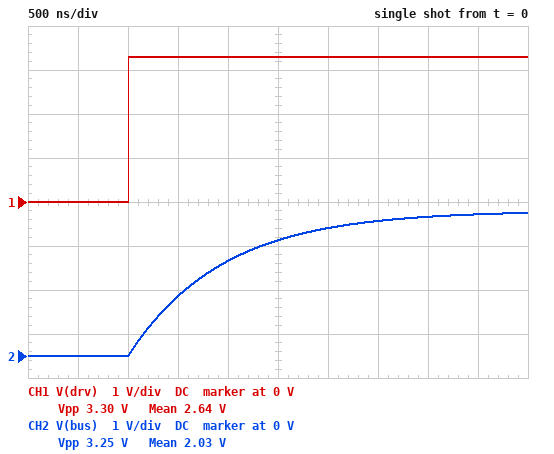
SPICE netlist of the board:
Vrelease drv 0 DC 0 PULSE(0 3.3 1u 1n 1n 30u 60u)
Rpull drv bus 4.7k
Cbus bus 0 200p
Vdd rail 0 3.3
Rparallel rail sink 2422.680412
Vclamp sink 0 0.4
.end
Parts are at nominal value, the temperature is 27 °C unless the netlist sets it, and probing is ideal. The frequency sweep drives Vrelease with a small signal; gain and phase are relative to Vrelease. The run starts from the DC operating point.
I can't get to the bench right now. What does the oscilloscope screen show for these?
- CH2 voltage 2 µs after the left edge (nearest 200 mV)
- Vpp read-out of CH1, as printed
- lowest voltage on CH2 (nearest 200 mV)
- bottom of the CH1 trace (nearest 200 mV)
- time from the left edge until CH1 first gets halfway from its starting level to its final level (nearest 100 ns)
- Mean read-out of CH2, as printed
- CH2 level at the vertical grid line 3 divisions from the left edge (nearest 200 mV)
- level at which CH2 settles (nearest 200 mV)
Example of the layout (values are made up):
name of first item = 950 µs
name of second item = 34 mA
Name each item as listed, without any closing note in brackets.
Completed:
CH2 voltage 2 µs after the left edge = 2.2 V
Vpp read-out of CH1, as printed = 3.30 V
lowest voltage on CH2 = 0 V
bottom of the CH1 trace = 0 V
time from the left edge until CH1 first gets halfway from its starting level to its final level = 1.0 µs
Mean read-out of CH2, as printed = 2.03 V
CH2 level at the vertical grid line 3 divisions from the left edge = 1.4 V
level at which CH2 settles = 3.2 V
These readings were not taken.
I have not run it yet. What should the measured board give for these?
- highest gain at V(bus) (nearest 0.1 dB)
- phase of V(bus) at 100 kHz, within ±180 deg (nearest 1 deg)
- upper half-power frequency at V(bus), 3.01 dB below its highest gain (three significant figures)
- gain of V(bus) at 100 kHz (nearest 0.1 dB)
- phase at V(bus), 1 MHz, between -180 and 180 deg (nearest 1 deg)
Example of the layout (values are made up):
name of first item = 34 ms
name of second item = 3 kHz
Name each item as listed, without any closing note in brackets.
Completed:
highest gain at V(bus) = 0 dB
phase of V(bus) at 100 kHz, within ±180 deg = -31 deg
upper half-power frequency at V(bus), 3.01 dB below its highest gain = 169 kHz
gain of V(bus) at 100 kHz = -1.3 dB
phase at V(bus), 1 MHz, between -180 and 180 deg = -80 deg
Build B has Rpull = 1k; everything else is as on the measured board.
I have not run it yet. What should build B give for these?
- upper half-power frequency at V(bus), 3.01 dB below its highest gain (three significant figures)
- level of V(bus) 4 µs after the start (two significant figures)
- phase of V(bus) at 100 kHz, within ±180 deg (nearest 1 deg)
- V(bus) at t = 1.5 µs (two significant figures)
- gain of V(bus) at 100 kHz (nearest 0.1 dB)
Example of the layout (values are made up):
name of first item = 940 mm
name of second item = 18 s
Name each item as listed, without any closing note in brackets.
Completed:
upper half-power frequency at V(bus), 3.01 dB below its highest gain = 796 kHz
level of V(bus) 4 µs after the start = 3.3 V
phase of V(bus) at 100 kHz, within ±180 deg = -7 deg
V(bus) at t = 1.5 µs = 3.0 V
gain of V(bus) at 100 kHz = -0.1 dB
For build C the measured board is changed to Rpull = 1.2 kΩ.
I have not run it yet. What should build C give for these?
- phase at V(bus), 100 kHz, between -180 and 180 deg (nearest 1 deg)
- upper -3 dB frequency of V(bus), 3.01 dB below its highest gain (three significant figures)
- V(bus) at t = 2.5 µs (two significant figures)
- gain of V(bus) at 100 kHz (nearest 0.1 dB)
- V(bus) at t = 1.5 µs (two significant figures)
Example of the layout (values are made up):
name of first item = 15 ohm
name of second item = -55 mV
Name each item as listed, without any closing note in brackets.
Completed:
phase at V(bus), 100 kHz, between -180 and 180 deg = -9 deg
upper -3 dB frequency of V(bus), 3.01 dB below its highest gain = 663 kHz
V(bus) at t = 2.5 µs = 3.3 V
gain of V(bus) at 100 kHz = -0.1 dB
V(bus) at t = 1.5 µs = 2.9 V
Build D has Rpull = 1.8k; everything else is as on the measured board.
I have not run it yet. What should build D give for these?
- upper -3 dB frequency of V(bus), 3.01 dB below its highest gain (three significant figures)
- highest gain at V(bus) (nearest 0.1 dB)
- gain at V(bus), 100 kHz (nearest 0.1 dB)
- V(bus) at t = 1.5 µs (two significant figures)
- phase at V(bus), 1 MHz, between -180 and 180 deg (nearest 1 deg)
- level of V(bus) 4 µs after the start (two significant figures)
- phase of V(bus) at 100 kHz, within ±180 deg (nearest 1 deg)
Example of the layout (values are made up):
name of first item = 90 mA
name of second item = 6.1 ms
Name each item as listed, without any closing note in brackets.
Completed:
upper -3 dB frequency of V(bus), 3.01 dB below its highest gain = 442 kHz
highest gain at V(bus) = 0 dB
gain at V(bus), 100 kHz = -0.2 dB
V(bus) at t = 1.5 µs = 2.5 V
phase at V(bus), 1 MHz, between -180 and 180 deg = -66 deg
level of V(bus) 4 µs after the start = 3.3 V
phase of V(bus) at 100 kHz, within ±180 deg = -13 deg
